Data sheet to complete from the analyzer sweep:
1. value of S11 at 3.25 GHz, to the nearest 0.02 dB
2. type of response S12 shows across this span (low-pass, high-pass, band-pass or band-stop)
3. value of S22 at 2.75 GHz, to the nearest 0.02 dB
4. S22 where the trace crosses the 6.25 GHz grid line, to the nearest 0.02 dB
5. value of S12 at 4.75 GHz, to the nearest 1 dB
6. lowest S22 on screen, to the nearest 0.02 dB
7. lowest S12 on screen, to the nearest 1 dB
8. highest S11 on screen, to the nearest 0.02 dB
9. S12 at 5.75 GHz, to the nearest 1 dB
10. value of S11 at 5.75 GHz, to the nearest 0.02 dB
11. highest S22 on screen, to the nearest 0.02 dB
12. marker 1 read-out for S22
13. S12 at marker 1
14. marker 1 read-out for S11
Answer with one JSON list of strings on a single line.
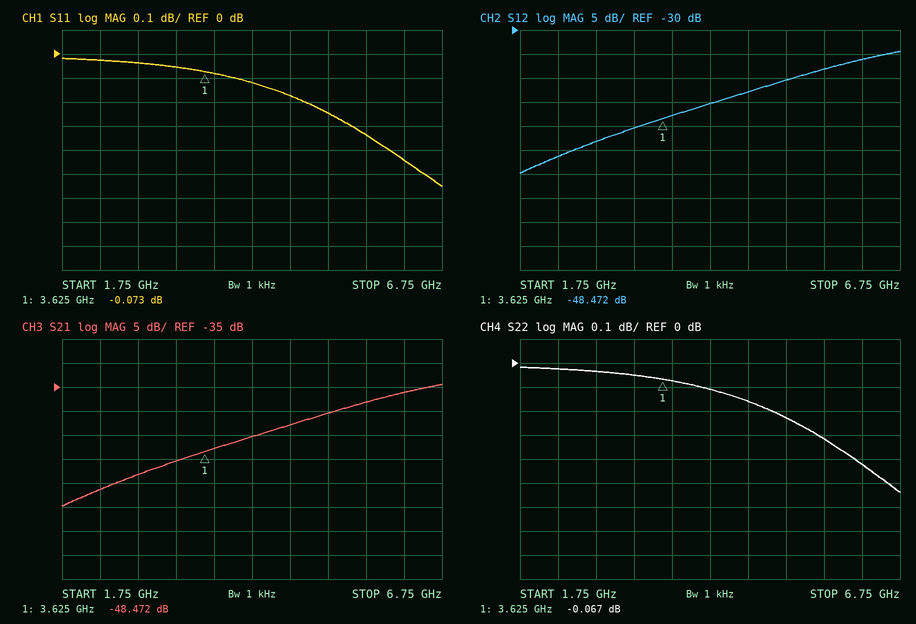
["-0.06 dB", "high-pass", "-0.04 dB", "-0.42 dB", "-43 dB", "-0.54 dB", "-60 dB", "-0.02 dB", "-38 dB", "-0.34 dB", "-0.02 dB", "-0.067 dB", "-48.472 dB", "-0.073 dB"]
